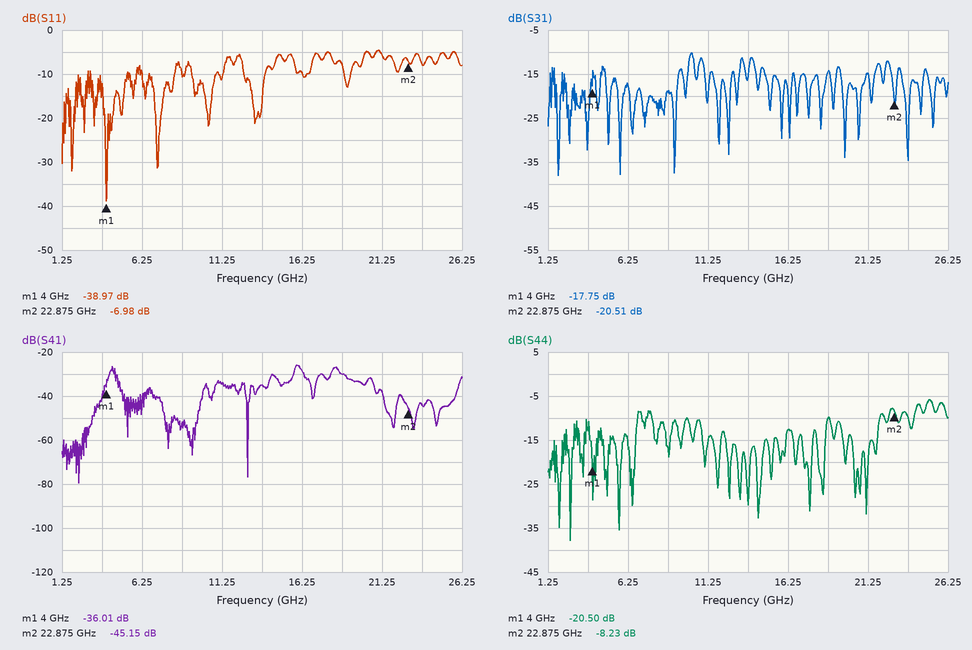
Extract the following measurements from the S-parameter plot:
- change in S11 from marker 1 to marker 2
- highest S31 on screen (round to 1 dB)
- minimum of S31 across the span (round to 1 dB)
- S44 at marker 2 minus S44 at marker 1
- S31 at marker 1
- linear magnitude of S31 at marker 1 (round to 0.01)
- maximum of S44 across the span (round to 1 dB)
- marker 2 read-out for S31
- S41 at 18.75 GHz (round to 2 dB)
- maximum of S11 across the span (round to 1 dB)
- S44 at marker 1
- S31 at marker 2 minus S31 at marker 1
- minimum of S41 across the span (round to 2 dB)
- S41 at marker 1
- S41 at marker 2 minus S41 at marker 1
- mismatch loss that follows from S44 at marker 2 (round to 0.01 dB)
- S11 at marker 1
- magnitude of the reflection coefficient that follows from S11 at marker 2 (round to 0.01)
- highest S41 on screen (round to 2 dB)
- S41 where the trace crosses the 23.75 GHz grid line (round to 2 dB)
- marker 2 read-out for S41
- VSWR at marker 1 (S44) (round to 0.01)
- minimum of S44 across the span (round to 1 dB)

31.99 dB
-10 dB
-38 dB
12.27 dB
-17.75 dB
0.13
-6 dB
-20.51 dB
-30 dB
-5 dB
-20.50 dB
-2.76 dB
-80 dB
-36.01 dB
-9.14 dB
0.71 dB
-38.97 dB
0.45
-26 dB
-44 dB
-45.15 dB
1.21
-38 dB
